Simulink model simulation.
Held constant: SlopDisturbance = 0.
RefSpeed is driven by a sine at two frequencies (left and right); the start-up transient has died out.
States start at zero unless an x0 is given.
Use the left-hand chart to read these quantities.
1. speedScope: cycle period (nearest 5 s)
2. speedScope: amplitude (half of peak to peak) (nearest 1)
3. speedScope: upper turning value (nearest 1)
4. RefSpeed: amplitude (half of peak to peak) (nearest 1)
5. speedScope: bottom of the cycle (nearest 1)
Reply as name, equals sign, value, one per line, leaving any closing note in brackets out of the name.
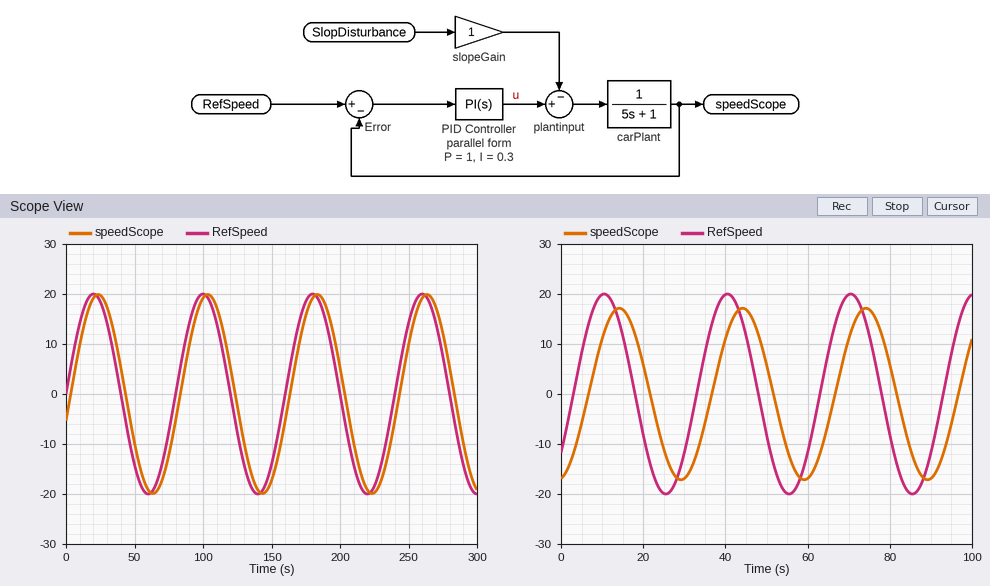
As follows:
speedScope: cycle period = 80 s
speedScope: amplitude (half of peak to peak) = 20
speedScope: upper turning value = 20
RefSpeed: amplitude (half of peak to peak) = 20
speedScope: bottom of the cycle = -20
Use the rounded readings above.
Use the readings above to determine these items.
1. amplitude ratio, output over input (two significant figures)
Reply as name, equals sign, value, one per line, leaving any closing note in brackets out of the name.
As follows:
amplitude ratio, output over input = 1.0
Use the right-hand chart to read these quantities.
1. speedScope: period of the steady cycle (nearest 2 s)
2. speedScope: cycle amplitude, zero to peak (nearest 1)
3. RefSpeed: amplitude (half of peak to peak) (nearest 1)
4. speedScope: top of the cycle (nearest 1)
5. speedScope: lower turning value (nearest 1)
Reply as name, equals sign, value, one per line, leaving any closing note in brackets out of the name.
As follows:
speedScope: period of the steady cycle = 30 s
speedScope: cycle amplitude, zero to peak = 17
RefSpeed: amplitude (half of peak to peak) = 20
speedScope: top of the cycle = 17
speedScope: lower turning value = -17
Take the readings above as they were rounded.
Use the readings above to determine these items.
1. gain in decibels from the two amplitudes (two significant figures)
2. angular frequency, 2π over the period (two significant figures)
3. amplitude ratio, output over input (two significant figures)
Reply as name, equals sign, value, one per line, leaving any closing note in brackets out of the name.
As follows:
gain in decibels from the two amplitudes = -1.4 dB
angular frequency, 2π over the period = 0.21 rad/s
amplitude ratio, output over input = 0.85
